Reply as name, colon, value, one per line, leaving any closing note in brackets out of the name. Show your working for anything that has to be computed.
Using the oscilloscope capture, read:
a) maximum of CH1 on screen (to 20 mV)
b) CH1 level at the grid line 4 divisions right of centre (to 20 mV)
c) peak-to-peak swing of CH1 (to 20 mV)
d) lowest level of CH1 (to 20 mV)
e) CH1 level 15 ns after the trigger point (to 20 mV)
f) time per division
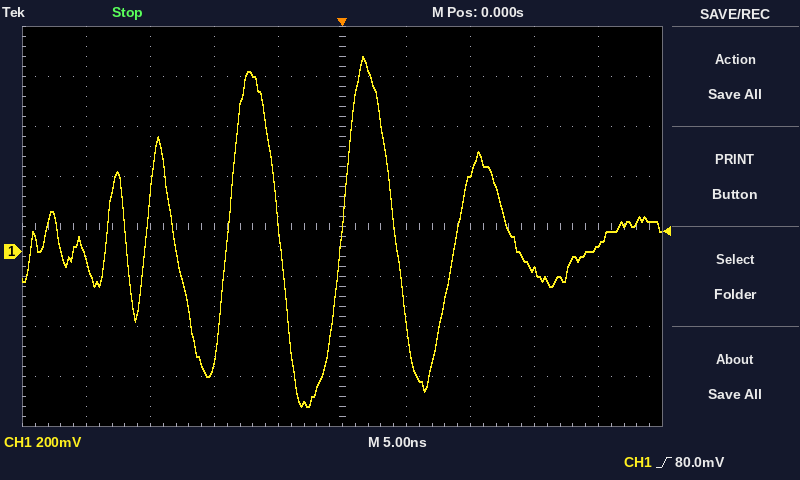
maximum of CH1 on screen: 780 mV
CH1 level at the grid line 4 divisions right of centre: 20 mV
peak-to-peak swing of CH1: 780 mV − (-620 mV) = 1.40 V
lowest level of CH1: -620 mV
CH1 level 15 ns after the trigger point: -80 mV
time per division: 5 ns
